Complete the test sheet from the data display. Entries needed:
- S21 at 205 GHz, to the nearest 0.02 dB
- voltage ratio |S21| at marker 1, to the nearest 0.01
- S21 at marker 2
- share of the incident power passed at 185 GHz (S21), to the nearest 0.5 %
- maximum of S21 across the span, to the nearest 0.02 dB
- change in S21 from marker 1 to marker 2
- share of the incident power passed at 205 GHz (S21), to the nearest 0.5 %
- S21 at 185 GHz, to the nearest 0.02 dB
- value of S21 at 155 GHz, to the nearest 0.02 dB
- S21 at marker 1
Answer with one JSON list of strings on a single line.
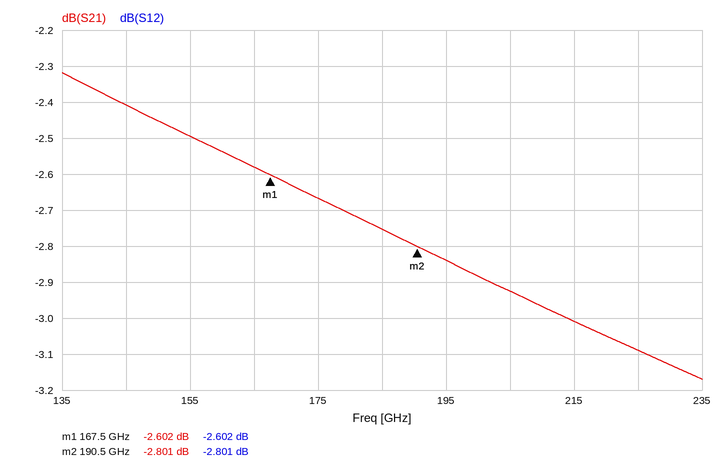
["-2.92 dB", "0.74", "-2.801 dB", "53.0 %", "-2.32 dB", "-0.199 dB", "51.0 %", "-2.76 dB", "-2.50 dB", "-2.602 dB"]
